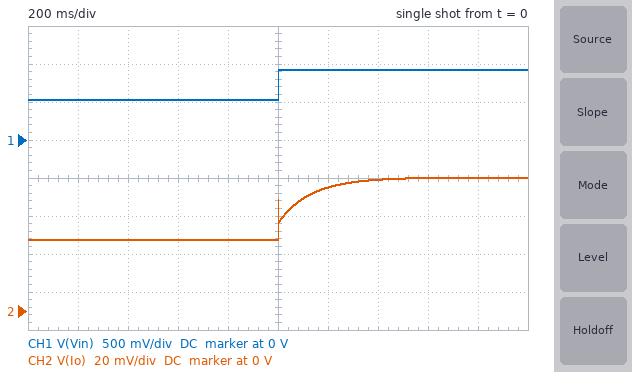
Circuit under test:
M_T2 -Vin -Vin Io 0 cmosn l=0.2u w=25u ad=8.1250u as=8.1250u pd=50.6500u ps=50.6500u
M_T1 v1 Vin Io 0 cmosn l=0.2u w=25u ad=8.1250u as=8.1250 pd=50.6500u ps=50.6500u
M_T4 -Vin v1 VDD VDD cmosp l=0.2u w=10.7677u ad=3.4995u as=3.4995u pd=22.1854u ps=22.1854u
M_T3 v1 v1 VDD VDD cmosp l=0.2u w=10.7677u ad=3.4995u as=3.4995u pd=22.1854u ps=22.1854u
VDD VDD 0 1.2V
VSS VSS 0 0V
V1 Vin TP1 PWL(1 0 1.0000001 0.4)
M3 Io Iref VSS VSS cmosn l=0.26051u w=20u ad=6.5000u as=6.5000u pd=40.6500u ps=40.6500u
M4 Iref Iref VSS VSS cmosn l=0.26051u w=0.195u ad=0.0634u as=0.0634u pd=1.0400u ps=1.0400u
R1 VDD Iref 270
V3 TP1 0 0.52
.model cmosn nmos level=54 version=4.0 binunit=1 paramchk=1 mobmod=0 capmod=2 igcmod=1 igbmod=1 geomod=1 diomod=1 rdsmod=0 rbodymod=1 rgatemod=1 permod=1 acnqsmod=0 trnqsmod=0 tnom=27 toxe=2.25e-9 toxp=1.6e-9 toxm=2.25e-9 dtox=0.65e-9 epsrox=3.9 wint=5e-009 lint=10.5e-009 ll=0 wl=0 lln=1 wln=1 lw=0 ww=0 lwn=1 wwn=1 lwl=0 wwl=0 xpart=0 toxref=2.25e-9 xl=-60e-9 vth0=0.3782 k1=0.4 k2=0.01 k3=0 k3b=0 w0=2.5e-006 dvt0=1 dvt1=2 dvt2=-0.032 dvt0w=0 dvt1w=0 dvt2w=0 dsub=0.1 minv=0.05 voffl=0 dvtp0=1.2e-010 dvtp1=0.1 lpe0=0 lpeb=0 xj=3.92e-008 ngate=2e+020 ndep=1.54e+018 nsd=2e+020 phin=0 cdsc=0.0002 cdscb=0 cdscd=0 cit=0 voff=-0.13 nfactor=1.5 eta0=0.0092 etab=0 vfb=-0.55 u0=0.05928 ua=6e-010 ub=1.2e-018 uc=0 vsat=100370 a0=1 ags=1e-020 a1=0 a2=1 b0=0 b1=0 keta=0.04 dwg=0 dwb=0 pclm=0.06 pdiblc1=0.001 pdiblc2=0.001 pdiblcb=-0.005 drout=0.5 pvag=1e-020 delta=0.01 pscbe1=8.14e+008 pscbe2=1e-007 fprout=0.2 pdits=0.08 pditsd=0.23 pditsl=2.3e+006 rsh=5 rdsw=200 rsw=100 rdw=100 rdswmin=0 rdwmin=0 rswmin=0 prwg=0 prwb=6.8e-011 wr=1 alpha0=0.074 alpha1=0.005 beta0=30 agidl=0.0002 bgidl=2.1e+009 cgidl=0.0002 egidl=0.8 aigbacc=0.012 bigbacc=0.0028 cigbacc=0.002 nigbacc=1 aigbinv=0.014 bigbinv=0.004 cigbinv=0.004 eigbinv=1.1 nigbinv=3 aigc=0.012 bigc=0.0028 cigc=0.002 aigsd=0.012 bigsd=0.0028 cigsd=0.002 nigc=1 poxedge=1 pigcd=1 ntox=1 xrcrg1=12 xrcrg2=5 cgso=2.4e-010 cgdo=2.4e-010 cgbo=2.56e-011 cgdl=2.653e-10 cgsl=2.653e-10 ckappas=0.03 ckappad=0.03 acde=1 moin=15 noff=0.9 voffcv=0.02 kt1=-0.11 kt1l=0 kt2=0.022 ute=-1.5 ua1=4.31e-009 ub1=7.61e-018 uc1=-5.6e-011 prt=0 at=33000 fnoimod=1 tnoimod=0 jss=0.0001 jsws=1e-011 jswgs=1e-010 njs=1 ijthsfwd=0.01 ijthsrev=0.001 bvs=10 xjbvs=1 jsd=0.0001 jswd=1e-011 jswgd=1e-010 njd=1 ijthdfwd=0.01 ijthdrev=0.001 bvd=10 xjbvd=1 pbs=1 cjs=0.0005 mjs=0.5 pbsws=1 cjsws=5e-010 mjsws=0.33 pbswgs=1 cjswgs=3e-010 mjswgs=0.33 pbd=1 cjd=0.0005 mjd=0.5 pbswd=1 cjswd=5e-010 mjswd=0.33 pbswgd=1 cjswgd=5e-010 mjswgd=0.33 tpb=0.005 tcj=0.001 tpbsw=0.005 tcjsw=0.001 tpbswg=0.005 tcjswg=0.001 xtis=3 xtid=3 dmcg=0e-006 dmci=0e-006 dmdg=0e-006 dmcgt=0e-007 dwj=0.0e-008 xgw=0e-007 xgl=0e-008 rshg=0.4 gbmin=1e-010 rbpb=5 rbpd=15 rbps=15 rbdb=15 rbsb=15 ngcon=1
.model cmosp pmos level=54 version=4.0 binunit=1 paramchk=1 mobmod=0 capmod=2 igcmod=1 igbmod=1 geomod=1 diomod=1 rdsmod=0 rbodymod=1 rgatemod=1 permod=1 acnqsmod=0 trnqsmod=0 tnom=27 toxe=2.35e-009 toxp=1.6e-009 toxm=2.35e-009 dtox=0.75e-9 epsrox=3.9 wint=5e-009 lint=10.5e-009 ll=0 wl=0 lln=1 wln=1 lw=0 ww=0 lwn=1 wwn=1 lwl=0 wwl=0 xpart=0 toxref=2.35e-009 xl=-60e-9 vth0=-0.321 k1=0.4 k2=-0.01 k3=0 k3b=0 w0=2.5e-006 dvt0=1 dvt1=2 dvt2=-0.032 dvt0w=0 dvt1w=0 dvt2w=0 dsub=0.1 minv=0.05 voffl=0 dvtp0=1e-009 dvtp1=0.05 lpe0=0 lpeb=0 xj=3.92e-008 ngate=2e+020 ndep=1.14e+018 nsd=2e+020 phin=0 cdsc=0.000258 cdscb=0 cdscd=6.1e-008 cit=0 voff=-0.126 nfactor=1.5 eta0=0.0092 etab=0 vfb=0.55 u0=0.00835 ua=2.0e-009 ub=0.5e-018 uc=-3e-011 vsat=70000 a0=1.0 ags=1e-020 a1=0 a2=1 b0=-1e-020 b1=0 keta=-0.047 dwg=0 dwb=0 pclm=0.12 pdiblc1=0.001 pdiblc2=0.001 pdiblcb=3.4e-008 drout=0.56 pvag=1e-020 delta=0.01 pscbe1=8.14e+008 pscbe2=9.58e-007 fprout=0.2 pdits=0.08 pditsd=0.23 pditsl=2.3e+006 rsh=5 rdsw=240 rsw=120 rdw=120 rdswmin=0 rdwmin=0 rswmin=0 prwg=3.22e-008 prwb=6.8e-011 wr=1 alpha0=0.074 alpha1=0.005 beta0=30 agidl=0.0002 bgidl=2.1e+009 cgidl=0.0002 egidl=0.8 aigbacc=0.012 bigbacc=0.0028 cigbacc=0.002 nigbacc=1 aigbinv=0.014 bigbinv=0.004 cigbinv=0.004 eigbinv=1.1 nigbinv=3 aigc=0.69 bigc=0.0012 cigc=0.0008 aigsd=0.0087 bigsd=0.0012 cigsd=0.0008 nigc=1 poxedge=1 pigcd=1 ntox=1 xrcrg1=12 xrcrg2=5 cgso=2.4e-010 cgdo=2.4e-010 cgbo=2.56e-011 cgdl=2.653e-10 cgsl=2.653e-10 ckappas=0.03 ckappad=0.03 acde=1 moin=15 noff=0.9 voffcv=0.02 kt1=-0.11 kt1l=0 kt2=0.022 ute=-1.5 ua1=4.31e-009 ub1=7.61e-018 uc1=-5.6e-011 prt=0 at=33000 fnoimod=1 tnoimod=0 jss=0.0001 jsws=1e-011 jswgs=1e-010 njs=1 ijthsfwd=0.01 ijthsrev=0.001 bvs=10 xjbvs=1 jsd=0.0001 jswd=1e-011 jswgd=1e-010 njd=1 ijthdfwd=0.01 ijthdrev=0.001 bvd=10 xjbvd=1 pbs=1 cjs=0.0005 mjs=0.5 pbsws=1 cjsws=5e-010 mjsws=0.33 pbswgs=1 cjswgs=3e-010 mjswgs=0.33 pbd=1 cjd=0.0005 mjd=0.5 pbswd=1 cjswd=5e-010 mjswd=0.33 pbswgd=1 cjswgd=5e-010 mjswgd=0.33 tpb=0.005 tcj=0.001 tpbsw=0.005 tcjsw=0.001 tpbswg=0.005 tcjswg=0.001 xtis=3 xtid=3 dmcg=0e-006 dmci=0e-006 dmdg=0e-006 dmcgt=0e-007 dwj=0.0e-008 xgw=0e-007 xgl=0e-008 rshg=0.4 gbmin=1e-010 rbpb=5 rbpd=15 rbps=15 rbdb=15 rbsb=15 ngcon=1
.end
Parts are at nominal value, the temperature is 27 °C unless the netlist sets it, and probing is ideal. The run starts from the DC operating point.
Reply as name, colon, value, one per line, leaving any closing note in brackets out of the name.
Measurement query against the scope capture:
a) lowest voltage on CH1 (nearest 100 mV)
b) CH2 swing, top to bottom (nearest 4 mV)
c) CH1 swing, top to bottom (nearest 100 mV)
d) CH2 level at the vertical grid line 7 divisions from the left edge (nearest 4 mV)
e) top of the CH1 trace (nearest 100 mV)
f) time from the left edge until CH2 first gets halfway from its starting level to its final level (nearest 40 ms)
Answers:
lowest voltage on CH1: 500 mV
CH2 swing, top to bottom: 32 mV
CH1 swing, top to bottom: 400 mV
CH2 level at the vertical grid line 7 divisions from the left edge: 68 mV
top of the CH1 trace: 900 mV
time from the left edge until CH2 first gets halfway from its starting level to its final level: 1.04 s
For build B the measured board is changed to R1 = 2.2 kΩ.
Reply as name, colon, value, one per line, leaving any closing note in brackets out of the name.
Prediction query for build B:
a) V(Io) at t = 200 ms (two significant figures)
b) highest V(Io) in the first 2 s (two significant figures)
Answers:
V(Io) at t = 200 ms: 39 mV
highest V(Io) in the first 2 s: 76 mV
